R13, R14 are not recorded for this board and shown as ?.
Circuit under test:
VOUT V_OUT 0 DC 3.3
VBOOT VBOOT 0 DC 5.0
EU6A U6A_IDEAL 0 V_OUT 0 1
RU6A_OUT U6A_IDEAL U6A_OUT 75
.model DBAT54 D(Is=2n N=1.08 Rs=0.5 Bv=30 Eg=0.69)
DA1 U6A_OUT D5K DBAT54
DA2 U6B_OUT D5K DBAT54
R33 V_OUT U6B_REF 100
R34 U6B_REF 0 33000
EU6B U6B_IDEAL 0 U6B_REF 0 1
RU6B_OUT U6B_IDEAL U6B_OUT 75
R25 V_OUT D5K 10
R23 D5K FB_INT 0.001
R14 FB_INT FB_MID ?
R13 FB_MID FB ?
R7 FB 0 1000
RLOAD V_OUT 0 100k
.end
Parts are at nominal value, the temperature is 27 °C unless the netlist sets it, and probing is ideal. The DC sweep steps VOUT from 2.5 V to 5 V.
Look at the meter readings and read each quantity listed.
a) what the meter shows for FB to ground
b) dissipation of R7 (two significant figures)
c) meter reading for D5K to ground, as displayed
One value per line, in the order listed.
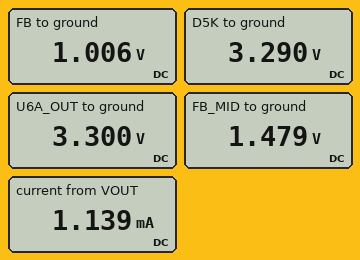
1.006 V
1.0 mW
3.290 V
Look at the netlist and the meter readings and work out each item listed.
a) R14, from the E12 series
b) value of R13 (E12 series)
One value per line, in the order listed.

1.8 kΩ
470 Ω
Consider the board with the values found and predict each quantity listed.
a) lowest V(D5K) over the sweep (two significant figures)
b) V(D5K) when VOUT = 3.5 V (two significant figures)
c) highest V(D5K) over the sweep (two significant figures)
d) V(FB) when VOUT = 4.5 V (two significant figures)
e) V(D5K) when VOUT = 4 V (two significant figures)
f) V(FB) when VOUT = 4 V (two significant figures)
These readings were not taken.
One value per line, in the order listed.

2.5 V
3.5 V
5.0 V
1.4 V
4.0 V
1.2 V
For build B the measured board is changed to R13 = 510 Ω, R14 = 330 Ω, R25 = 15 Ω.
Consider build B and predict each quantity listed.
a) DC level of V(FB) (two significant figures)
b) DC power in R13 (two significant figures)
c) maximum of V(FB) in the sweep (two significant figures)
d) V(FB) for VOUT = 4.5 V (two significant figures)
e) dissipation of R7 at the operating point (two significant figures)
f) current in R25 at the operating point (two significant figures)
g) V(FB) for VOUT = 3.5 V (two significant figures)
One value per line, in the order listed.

1.8 V
1.6 mW
2.7 V
2.4 V
3.2 mW
1.8 mA
1.9 V
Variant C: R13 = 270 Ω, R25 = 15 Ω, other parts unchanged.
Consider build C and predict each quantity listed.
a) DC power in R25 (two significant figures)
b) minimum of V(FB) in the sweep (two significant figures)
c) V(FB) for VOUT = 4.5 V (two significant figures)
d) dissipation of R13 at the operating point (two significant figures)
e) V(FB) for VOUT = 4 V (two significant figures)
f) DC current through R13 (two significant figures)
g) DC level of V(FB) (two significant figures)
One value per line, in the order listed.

17 µW
810 mV
1.5 V
310 µW
1.3 V
1.1 mA
1.1 V
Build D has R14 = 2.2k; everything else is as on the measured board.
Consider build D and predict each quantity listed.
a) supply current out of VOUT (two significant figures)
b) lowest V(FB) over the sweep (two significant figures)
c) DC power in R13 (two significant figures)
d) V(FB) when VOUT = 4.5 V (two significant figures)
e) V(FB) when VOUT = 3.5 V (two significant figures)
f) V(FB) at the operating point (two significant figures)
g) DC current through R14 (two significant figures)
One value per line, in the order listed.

1.0 mA
680 mV
380 µW
1.2 V
950 mV
900 mV
900 µA
